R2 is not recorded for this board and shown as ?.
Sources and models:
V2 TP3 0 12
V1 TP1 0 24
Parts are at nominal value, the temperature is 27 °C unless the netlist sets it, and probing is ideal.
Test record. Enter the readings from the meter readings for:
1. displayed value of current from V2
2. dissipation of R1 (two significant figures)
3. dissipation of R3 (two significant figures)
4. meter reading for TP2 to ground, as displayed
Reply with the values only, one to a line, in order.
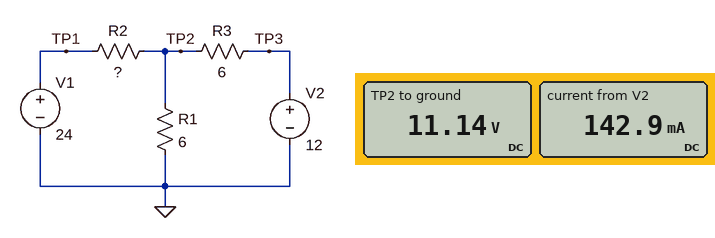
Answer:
142.9 mA
21 W
120 mW
11.14 V
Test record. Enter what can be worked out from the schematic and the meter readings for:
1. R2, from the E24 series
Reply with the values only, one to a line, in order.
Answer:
7.5 Ω
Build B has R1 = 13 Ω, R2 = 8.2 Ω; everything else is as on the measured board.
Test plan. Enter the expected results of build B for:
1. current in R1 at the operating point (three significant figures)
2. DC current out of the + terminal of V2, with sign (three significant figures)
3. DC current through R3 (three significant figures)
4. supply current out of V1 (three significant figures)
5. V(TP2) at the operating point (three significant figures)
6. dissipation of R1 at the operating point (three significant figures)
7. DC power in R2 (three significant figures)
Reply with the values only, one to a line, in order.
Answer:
1.04 A
-246 mA
246 mA
1.28 A
13.5 V
14.0 W
13.5 W
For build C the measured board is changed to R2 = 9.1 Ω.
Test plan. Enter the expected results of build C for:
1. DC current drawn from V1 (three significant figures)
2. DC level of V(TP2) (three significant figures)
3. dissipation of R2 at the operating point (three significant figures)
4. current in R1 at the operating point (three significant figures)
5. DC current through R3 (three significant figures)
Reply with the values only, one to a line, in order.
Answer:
1.49 A
10.5 V
20.1 W
1.74 A
256 mA
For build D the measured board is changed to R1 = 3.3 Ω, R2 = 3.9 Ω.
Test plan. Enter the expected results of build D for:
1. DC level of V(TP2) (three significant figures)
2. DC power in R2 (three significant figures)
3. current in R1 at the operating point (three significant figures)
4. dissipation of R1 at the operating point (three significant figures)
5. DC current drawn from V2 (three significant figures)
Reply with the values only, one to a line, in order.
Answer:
11.2 V
41.8 W
3.40 A
38.2 W
128 mA
